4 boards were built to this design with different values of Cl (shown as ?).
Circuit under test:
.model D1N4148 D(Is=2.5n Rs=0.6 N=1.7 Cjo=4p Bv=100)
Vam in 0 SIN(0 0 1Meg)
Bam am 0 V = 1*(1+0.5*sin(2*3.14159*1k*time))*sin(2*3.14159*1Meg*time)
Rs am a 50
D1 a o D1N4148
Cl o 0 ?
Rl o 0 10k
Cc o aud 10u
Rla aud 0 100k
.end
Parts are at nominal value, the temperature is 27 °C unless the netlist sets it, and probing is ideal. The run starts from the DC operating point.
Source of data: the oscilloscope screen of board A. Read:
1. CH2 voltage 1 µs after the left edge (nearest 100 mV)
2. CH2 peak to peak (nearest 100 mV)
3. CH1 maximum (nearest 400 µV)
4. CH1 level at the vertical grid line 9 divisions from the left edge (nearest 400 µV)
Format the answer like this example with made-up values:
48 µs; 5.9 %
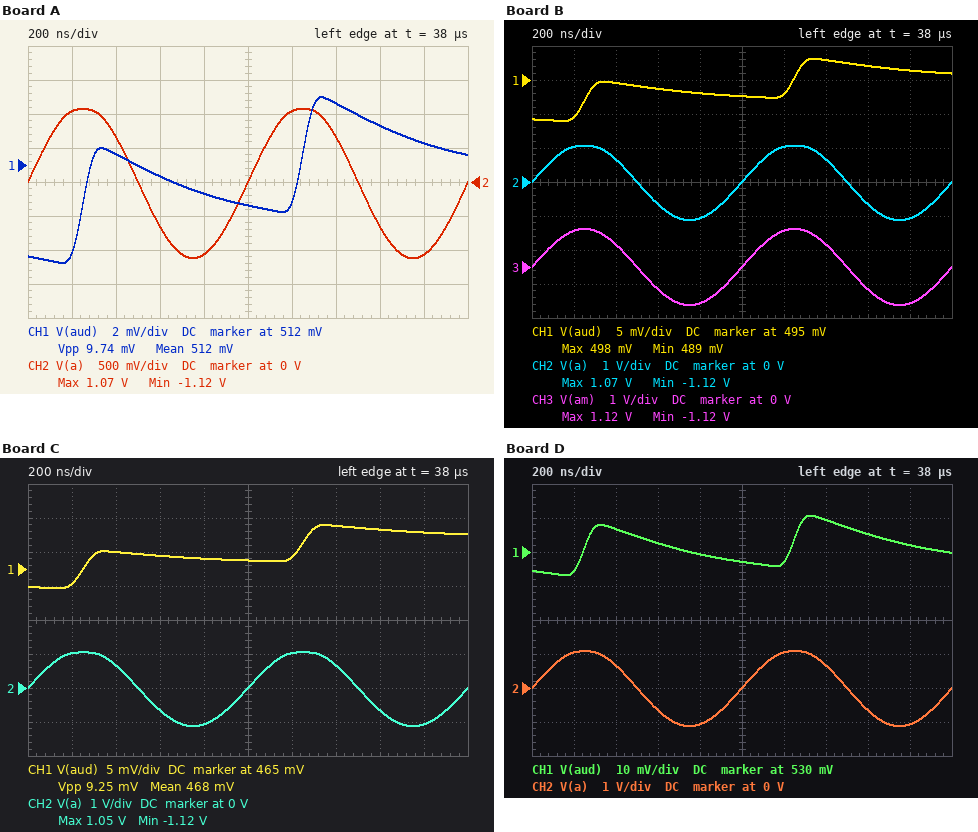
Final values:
0 V; 2.2 V; 516.0 mV; 513.2 mV
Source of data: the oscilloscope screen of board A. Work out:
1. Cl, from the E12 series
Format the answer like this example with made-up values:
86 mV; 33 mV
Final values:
12 nF
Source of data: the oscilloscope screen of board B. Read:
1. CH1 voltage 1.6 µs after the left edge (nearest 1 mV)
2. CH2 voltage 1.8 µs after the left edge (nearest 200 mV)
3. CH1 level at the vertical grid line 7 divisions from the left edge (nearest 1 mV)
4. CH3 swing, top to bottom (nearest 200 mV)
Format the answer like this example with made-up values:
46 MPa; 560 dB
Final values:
497 mV; -1.0 V; 498 mV; 2.2 V
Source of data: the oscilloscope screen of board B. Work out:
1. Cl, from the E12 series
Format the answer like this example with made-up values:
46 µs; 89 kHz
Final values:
18 nF
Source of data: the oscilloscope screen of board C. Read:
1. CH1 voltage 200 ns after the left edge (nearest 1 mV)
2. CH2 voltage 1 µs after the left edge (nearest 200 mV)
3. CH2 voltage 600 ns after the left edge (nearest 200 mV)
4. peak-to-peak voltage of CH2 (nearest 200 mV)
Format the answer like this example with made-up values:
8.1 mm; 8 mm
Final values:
463 mV; 0 V; -600 mV; 2.2 V
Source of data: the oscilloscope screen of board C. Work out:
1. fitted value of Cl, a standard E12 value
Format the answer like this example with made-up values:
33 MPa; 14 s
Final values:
27 nF
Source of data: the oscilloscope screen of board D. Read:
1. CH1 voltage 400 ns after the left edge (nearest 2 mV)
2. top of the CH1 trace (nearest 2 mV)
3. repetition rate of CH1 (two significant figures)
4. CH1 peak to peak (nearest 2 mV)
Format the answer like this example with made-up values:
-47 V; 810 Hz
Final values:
536 mV; 540 mV; 1.0 MHz; 18 mV
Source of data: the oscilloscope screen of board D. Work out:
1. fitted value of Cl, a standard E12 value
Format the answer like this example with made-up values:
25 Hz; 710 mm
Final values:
3.9 nF
